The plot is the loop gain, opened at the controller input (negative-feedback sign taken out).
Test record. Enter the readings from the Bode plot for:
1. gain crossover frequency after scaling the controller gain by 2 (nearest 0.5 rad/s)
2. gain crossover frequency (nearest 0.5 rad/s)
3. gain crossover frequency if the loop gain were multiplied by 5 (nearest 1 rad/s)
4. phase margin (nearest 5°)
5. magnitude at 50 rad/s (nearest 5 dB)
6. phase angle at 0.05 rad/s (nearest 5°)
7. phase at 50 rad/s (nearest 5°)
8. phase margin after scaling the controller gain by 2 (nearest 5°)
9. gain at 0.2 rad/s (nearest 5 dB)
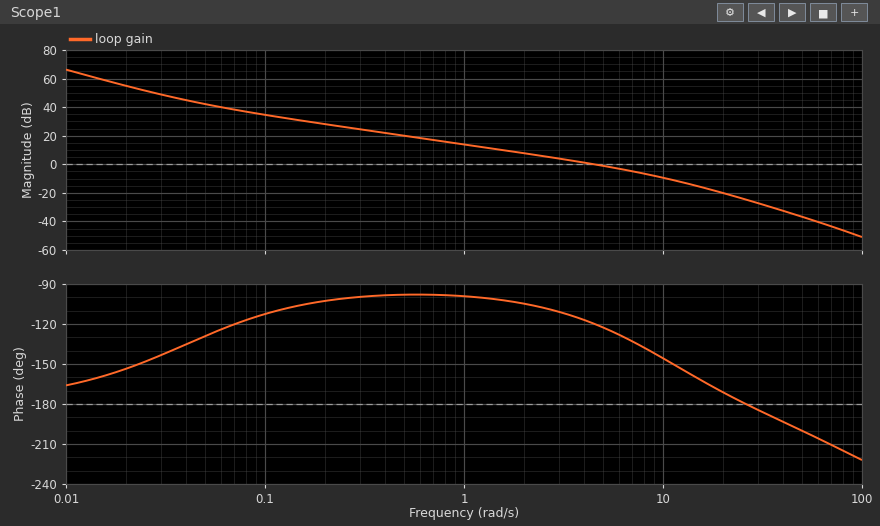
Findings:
7.5 rad/s
4.5 rad/s
14 rad/s
60°
-35 dB
-130°
-200°
45°
30 dB
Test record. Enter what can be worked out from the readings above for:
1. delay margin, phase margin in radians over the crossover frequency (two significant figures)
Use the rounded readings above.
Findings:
0.23 s
